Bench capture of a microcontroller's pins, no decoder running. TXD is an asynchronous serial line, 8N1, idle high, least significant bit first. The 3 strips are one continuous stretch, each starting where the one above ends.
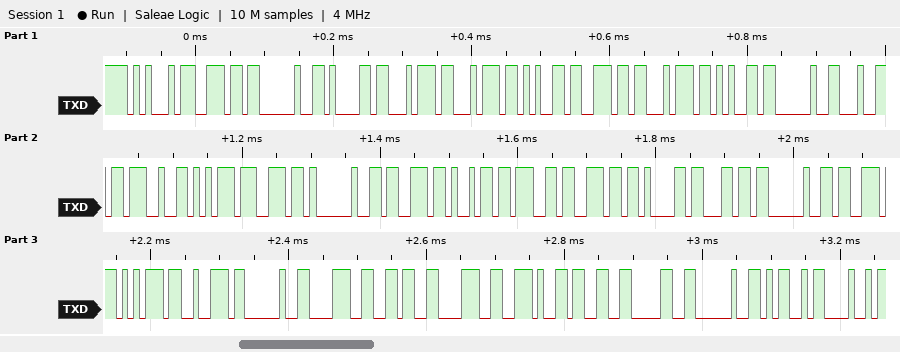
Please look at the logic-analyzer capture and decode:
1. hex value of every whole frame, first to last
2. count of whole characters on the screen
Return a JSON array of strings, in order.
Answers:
["45 6E 20 61 74 74 65 6E 74 65 20 64 27 75 6E 20 73 69 67 6E 61 6C 20 73 75 72 20 38 36 38 2E 33 30 20 4D 48", "36"]
